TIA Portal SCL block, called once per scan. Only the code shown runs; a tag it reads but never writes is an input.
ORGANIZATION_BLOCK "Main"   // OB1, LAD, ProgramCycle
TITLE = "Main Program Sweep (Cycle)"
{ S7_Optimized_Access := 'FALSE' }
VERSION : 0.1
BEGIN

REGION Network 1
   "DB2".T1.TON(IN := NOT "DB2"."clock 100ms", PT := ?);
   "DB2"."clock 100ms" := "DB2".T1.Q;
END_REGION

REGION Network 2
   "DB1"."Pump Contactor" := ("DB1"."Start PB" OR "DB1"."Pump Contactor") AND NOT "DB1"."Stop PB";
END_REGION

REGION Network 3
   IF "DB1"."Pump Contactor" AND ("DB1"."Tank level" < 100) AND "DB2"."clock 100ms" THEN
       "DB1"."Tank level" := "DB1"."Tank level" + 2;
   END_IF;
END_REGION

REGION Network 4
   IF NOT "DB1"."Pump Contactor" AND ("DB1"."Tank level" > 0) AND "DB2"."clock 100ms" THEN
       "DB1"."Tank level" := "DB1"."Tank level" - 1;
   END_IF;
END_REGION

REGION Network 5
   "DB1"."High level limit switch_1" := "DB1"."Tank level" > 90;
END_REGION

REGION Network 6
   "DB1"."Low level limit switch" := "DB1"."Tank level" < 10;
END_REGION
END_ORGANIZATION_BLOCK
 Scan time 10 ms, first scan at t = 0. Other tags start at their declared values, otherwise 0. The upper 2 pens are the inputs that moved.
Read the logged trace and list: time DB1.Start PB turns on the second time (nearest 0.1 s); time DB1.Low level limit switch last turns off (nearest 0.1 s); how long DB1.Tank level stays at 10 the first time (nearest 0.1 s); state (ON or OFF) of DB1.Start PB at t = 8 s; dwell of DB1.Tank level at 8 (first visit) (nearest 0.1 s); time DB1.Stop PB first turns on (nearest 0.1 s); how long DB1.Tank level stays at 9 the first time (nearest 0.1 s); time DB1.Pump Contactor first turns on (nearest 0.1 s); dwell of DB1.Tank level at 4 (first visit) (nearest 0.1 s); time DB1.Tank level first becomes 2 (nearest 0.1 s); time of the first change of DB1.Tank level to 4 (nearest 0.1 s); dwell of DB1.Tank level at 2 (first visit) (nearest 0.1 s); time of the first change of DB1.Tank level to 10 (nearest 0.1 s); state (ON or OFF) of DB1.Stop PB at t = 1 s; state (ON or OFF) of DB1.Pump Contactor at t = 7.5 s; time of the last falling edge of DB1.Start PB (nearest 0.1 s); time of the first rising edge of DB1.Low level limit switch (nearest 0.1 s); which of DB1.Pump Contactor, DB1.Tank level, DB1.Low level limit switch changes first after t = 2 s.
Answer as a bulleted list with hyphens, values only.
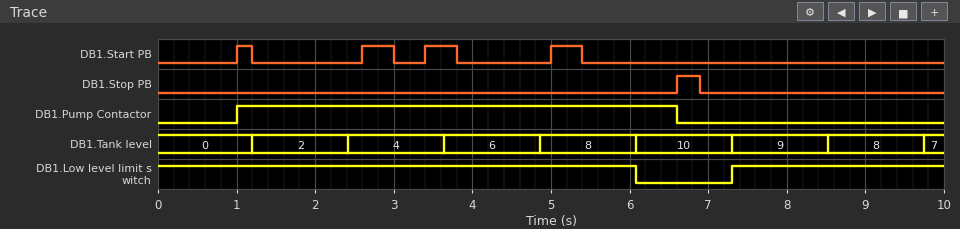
- 2.6 s
- 6.1 s
- 1.2 s
- OFF
- 1.2 s
- 6.6 s
- 1.2 s
- 1.0 s
- 1.2 s
- 1.2 s
- 2.4 s
- 1.2 s
- 6.1 s
- OFF
- OFF
- 5.4 s
- 7.3 s
- DB1.Tank level
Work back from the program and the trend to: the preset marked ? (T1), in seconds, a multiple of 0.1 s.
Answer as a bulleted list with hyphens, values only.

- 1.2 s
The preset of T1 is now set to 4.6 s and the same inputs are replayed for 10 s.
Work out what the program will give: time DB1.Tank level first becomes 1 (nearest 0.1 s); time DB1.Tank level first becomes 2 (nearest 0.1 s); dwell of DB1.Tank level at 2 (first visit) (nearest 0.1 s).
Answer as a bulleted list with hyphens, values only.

- 9.2 s
- 4.6 s
- 4.6 s
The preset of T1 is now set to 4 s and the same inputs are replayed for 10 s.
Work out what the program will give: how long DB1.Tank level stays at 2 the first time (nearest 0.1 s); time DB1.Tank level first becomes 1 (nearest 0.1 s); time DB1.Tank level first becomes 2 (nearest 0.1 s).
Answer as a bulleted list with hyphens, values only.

- 4.0 s
- 8.0 s
- 4.0 s
